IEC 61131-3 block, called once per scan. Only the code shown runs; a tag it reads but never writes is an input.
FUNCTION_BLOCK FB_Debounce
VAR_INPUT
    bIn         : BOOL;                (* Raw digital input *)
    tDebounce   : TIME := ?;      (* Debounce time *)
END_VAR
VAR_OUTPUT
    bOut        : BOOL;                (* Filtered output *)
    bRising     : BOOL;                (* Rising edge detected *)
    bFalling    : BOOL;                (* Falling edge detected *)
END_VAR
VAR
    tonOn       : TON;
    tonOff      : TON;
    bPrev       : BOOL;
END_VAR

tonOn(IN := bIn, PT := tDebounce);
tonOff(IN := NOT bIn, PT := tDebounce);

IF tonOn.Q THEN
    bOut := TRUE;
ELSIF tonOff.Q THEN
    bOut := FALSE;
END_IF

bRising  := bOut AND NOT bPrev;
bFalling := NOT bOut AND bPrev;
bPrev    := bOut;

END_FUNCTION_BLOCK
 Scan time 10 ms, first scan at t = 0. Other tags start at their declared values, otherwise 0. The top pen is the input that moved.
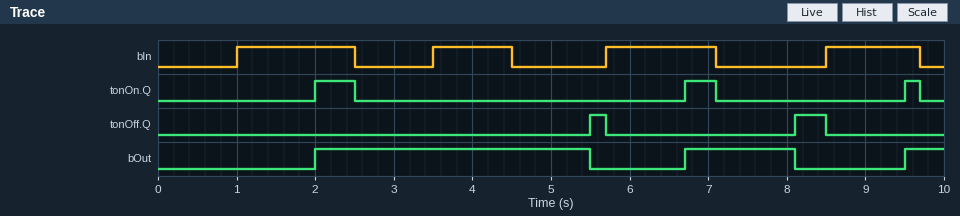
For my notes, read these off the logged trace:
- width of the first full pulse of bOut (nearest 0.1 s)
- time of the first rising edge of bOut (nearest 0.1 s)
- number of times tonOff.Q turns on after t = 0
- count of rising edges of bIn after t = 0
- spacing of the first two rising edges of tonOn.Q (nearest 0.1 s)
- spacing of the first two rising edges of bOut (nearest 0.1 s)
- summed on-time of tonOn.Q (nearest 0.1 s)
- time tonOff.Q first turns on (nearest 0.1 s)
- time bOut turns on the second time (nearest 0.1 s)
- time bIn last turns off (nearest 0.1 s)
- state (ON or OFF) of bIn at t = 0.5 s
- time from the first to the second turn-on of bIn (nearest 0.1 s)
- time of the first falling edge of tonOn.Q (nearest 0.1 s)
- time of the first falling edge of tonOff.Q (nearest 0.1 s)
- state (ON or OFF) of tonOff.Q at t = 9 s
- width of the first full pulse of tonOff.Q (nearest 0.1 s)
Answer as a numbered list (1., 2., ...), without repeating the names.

1. 3.5 s
2. 2.0 s
3. 2
4. 4
5. 4.7 s
6. 4.7 s
7. 1.1 s
8. 5.5 s
9. 6.7 s
10. 9.7 s
11. OFF
12. 2.5 s
13. 2.5 s
14. 5.7 s
15. OFF
16. 0.2 s
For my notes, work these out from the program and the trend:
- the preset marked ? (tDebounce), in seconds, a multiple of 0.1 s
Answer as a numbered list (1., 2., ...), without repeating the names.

1. 1.0 s
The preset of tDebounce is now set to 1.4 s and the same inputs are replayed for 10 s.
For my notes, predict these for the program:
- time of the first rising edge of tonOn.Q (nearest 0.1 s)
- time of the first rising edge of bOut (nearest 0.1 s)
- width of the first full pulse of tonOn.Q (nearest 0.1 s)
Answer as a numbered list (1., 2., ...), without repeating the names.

1. 2.4 s
2. 2.4 s
3. 0.1 s
